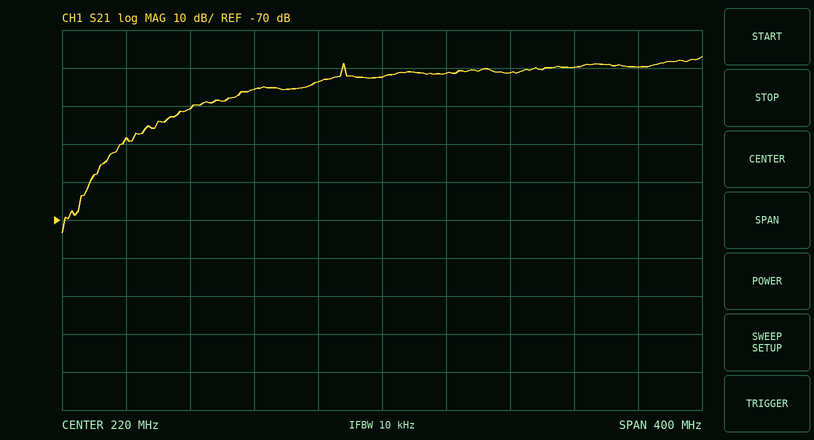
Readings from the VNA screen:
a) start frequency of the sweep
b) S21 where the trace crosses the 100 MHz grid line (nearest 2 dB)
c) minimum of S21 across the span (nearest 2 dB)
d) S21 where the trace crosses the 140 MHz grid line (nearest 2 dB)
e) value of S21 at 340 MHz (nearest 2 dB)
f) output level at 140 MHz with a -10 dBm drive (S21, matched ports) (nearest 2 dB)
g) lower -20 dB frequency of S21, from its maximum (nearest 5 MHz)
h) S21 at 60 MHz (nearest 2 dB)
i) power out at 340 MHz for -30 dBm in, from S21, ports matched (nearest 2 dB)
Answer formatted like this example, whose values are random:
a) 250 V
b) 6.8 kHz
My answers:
a) 20 MHz
b) -40 dB
c) -74 dB
d) -36 dB
e) -30 dB
f) -46 dBm
g) 70 MHz
h) -48 dB
i) -60 dBm
